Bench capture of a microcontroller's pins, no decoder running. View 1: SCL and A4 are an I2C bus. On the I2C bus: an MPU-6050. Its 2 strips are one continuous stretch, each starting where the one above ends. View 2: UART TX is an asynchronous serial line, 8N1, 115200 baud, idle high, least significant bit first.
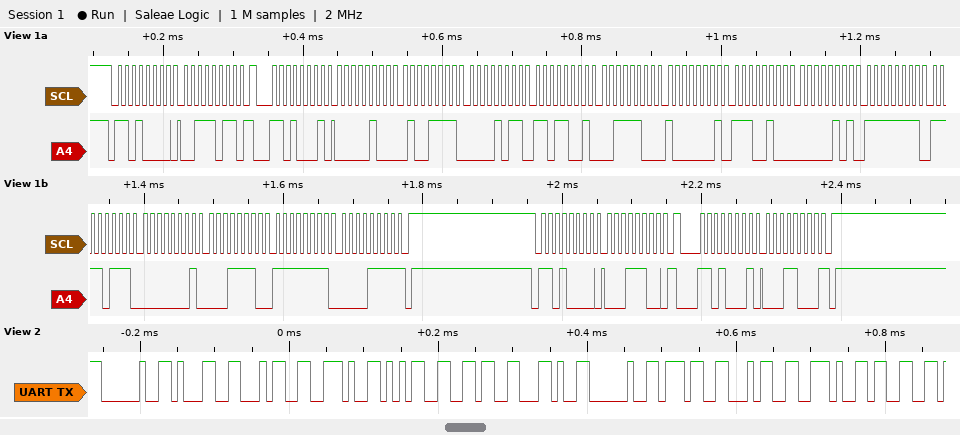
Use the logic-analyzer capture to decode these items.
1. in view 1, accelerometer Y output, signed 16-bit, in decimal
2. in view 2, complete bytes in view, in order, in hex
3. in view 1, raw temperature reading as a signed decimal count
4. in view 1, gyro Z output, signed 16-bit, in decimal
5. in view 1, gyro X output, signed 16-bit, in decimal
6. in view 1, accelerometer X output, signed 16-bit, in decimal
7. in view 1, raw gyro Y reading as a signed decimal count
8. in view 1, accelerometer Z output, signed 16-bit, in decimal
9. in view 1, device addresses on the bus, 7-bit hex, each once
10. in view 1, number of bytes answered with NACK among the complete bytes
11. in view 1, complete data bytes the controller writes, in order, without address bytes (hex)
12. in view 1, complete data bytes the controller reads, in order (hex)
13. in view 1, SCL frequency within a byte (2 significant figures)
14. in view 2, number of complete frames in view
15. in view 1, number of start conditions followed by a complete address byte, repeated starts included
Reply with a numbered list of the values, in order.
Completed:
1. 3033
2. 0x20 0x31 0x34 0x2E 0x35 0x36 0x2C 0x20 0x37 0x34 0x2E 0x33
3. -7163
4. -241
5. -9
6. 1103
7. 286
8. 15489
9. 0x68
10. 2
11. 3B 1C
12. 04 4F 0B D9 3C 81 E4 05 FF F7 01 1E FF 0F 18
13. 100 kHz
14. 12
15. 4
